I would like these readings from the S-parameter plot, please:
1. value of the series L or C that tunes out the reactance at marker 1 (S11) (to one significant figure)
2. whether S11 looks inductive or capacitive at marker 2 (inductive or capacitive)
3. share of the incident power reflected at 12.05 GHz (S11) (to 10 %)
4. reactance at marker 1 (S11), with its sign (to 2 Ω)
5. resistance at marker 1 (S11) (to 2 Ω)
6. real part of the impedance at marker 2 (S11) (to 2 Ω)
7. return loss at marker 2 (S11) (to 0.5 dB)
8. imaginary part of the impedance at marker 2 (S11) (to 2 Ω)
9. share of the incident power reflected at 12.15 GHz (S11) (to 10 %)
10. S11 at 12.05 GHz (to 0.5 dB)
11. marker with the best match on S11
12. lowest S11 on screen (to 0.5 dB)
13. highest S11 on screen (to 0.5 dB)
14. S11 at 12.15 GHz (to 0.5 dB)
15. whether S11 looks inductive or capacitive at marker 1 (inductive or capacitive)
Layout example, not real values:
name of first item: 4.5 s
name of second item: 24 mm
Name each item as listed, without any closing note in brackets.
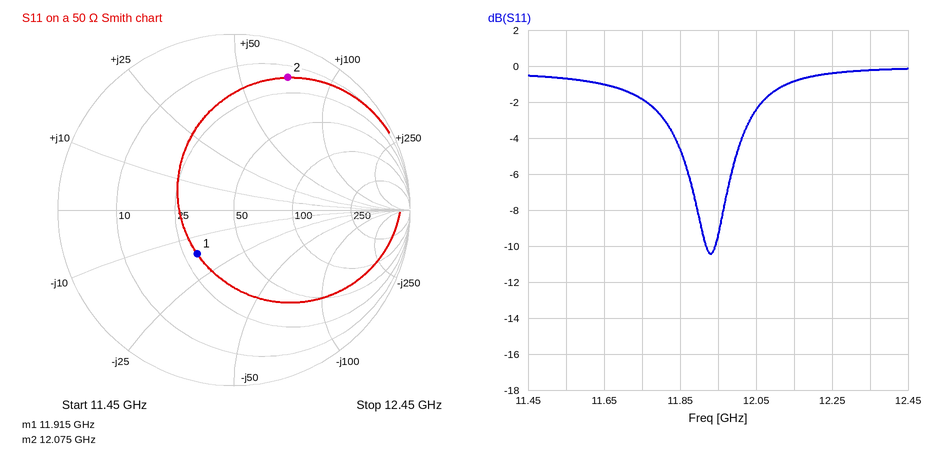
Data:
value of the series L or C that tunes out the reactance at marker 1 (S11): 200 pH
whether S11 looks inductive or capacitive at marker 2: inductive
share of the incident power reflected at 12.05 GHz (S11): 60 %
reactance at marker 1 (S11), with its sign: -16 Ω
resistance at marker 1 (S11): 30 Ω
real part of the impedance at marker 2 (S11): 16 Ω
return loss at marker 2 (S11): 2.0 dB
imaginary part of the impedance at marker 2 (S11): +72 Ω
share of the incident power reflected at 12.15 GHz (S11): 80 %
S11 at 12.05 GHz: -2.5 dB
marker with the best match on S11: marker 1
lowest S11 on screen: -10.5 dB
highest S11 on screen: 0.0 dB
S11 at 12.15 GHz: -1.0 dB
whether S11 looks inductive or capacitive at marker 1: capacitive
